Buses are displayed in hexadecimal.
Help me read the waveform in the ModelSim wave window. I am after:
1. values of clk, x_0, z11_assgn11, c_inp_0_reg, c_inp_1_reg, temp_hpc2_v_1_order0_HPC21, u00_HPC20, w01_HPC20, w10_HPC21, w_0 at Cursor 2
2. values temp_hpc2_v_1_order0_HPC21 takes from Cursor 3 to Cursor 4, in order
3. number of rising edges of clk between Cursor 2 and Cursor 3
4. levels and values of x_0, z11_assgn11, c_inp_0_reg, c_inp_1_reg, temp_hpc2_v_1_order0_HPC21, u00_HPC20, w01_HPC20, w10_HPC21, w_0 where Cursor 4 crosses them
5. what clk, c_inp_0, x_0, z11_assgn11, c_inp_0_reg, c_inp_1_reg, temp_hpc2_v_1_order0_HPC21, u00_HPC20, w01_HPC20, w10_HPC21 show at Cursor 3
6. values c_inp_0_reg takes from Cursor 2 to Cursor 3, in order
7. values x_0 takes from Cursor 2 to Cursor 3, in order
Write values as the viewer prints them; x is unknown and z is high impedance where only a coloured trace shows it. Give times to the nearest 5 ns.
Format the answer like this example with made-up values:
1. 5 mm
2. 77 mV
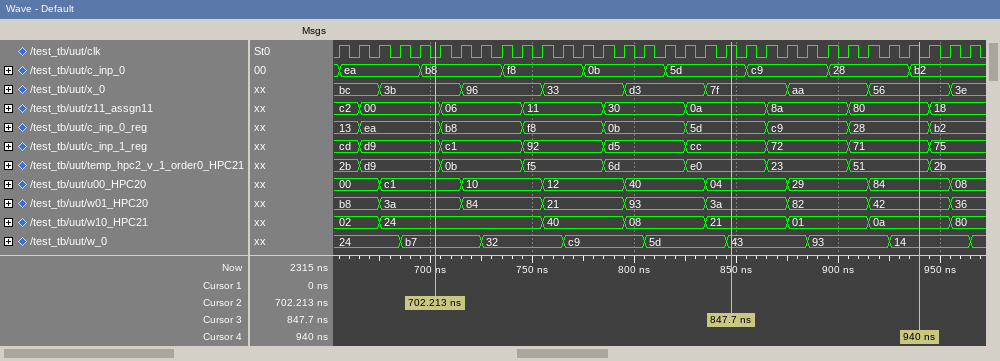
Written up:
1. clk=0, x_0=3b, z11_assgn11=00, c_inp_0_reg=ea, c_inp_1_reg=d9, temp_hpc2_v_1_order0_HPC21=d9, u00_HPC20=c1, w01_HPC20=3a, w10_HPC21=24, w_0=b7
2. e0, 23, 51
3. 15
4. x_0=56, z11_assgn11=80, c_inp_0_reg=28, c_inp_1_reg=71, temp_hpc2_v_1_order0_HPC21=51, u00_HPC20=84, w01_HPC20=42, w10_HPC21=0a, w_0=14
5. clk=1, c_inp_0=5d, x_0=7f, z11_assgn11=0a, c_inp_0_reg=5d, c_inp_1_reg=cc, temp_hpc2_v_1_order0_HPC21=e0, u00_HPC20=04, w01_HPC20=3a, w10_HPC21=21
6. ea, b8, f8, 0b, 5d
7. 3b, 96, 33, d3, 7f
